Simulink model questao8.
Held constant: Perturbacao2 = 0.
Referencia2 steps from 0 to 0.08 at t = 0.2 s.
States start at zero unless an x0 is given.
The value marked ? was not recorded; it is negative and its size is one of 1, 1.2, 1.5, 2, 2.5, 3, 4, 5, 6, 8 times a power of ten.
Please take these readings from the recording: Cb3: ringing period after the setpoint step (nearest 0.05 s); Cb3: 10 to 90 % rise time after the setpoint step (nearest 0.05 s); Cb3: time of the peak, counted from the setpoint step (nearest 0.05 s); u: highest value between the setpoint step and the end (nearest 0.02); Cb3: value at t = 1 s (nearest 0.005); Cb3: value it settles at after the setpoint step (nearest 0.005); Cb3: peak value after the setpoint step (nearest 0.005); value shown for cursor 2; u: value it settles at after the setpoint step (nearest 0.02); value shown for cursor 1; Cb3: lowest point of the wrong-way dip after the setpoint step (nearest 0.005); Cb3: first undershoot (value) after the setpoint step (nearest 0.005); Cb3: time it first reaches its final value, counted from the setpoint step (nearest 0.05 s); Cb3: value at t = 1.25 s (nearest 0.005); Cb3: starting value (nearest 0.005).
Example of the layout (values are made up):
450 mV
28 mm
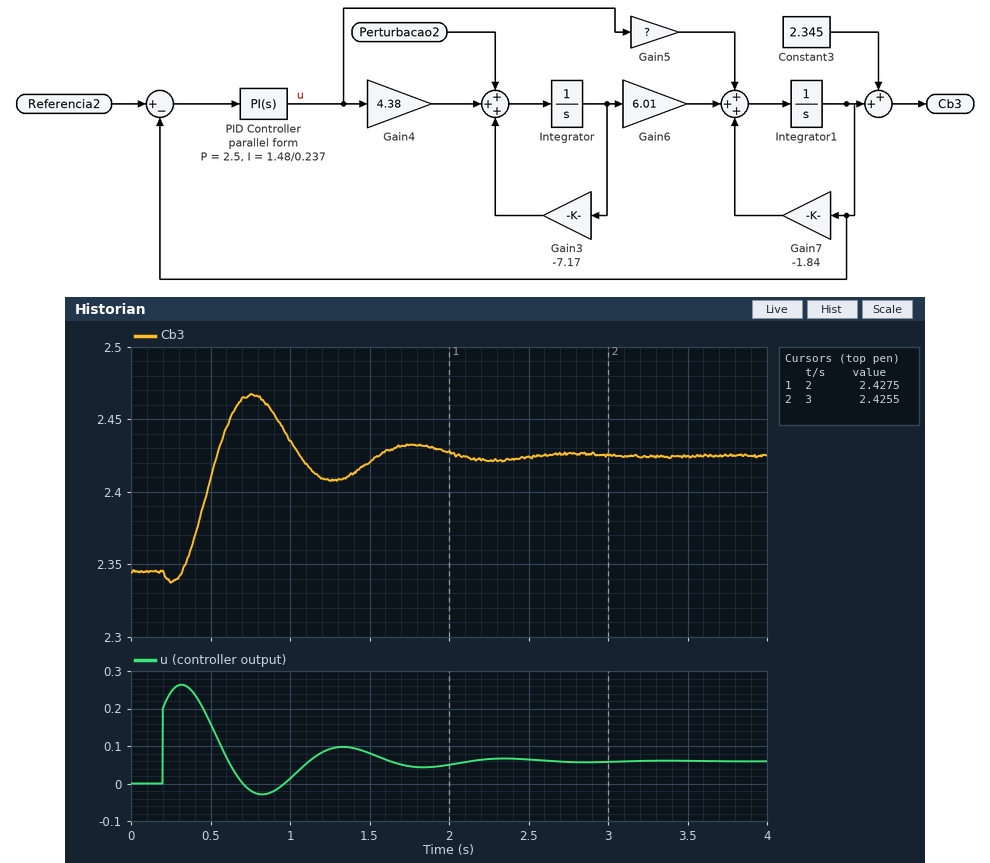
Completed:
1.00 s
0.15 s
0.55 s
0.26
2.435
2.425
2.465
2.4255
0.06
2.4275
2.340
2.410
0.35 s
2.410
2.345
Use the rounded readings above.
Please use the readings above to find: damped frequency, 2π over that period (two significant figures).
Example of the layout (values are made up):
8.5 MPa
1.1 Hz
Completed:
6.3 rad/s
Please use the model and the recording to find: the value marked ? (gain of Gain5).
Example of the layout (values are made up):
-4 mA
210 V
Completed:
-1.2
